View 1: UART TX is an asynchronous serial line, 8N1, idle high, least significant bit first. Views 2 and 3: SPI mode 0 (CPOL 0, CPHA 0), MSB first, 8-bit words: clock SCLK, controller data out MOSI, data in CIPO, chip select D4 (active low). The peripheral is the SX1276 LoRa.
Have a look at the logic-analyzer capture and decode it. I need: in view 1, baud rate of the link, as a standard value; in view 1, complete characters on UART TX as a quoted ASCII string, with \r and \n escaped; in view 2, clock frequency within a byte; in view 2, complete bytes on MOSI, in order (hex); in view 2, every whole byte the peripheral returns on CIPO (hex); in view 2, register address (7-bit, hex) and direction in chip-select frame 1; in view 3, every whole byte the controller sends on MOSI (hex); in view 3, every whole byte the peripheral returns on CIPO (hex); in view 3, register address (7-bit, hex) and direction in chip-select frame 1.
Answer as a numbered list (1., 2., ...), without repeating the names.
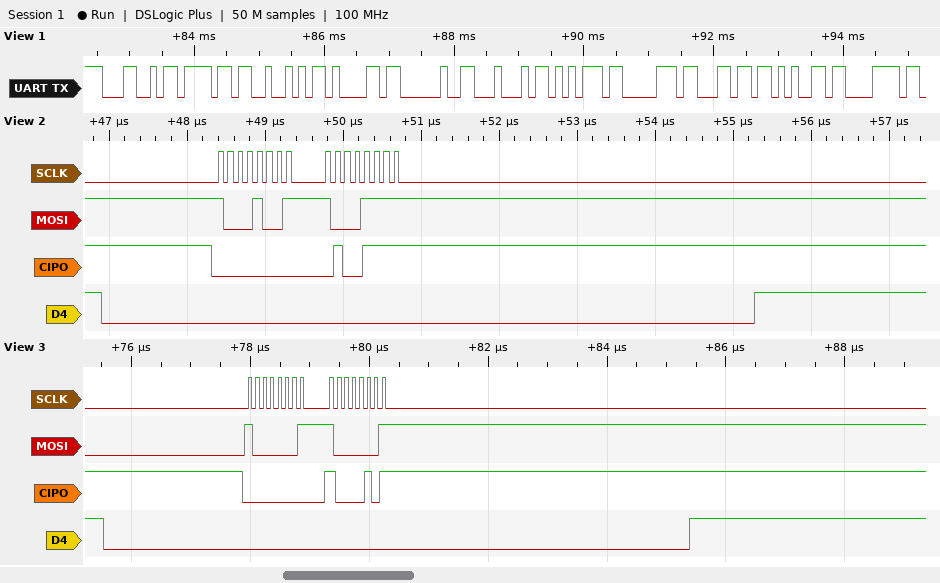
1. 9600 baud
2. "LoRa Duplex"
3. 8 MHz
4. 89 8F
5. 00 4F
6. 0x09 write
7. 81 81
8. 00 85
9. 0x01 write
